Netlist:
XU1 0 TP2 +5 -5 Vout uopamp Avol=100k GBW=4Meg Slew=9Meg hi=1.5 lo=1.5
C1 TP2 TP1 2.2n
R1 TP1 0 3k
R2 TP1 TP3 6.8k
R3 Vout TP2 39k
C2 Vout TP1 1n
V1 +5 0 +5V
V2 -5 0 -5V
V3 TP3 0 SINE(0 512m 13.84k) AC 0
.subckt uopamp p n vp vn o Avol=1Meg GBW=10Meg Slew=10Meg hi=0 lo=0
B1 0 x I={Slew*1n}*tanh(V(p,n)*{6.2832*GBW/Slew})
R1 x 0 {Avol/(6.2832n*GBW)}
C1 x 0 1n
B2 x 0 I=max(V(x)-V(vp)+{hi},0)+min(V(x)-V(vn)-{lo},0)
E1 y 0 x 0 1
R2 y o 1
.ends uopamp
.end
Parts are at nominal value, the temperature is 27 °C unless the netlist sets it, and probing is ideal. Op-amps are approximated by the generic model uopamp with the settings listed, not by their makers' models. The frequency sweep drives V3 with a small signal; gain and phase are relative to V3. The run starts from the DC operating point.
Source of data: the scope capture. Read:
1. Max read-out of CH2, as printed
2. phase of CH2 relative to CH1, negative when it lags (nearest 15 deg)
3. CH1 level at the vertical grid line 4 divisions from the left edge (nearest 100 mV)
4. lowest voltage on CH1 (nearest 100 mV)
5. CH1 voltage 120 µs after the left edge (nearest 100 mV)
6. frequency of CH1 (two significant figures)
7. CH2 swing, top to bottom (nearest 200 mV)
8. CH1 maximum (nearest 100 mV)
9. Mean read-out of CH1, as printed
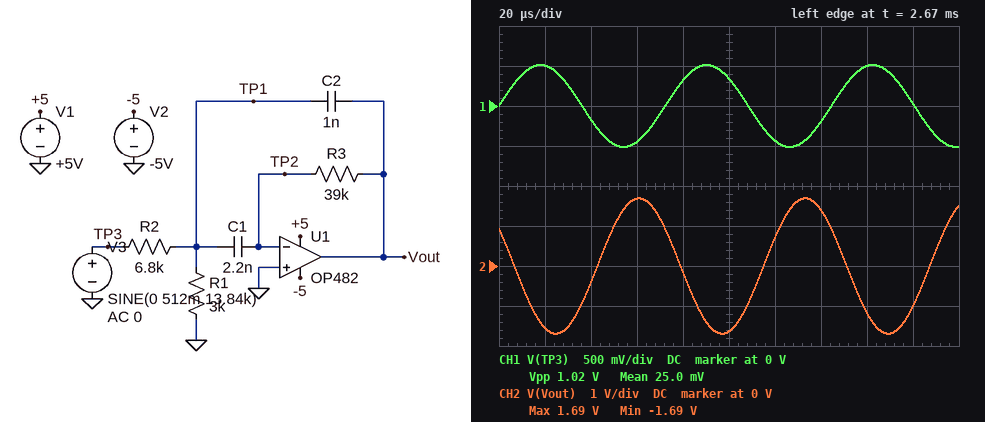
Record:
1.69 V
150 deg
300 mV
-500 mV
-400 mV
14 kHz
3.4 V
500 mV
25.0 mV
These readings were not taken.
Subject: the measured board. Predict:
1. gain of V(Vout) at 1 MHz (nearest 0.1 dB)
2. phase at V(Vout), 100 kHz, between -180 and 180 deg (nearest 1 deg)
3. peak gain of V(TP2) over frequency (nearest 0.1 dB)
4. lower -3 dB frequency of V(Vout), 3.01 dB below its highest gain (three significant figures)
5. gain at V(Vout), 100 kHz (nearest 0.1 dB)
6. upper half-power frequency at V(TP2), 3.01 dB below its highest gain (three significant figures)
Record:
-33.0 dB
92 deg
-38.4 dB
9.24 kHz
-12.7 dB
18.7 kHz
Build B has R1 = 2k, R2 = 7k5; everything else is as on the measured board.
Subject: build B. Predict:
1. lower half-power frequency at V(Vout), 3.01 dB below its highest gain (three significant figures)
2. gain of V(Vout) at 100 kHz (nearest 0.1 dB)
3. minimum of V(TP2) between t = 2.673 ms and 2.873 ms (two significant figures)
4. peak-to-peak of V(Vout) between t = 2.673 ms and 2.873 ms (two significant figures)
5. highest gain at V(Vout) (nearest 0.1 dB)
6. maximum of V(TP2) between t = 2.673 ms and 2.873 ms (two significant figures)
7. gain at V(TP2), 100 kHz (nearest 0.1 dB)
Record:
10.9 kHz
-13.5 dB
-6.3 mV
3.6 V
11.1 dB
6.3 mV
-45.6 dB
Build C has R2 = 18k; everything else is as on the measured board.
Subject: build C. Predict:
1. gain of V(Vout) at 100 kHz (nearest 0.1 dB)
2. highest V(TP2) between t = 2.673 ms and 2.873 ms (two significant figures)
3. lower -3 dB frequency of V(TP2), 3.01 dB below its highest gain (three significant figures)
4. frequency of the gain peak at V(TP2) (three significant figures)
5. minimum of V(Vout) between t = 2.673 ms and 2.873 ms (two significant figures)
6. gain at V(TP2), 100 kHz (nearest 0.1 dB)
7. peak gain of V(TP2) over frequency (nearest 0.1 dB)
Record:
-21.1 dB
1.9 mV
9.06 kHz
11.5 kHz
-550 mV
-53.2 dB
-47.7 dB
